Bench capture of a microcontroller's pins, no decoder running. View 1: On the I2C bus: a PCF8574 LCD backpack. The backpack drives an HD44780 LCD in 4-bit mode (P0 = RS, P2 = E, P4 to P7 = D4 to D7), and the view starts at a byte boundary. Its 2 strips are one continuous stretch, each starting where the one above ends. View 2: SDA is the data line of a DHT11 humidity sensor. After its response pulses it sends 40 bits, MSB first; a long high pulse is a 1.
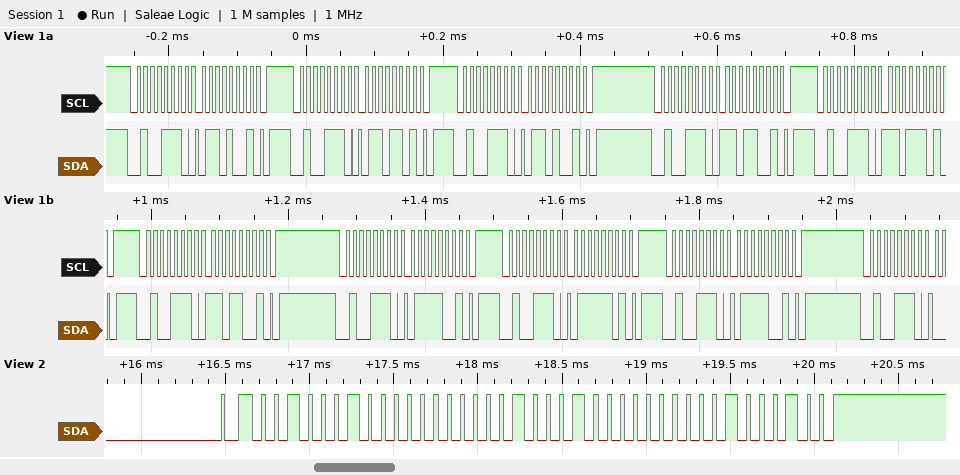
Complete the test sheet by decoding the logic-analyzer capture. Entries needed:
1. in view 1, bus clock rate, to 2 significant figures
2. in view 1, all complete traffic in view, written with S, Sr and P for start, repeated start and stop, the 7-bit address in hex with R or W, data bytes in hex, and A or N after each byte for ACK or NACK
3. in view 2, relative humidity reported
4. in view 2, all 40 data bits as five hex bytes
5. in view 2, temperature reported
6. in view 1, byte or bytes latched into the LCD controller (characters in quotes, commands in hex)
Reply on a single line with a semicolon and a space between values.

100 kHz; S 27W A 69 A P S 27W A 6D A P S 27W A 69 A P S 27W A D9 A P S 27W A DD A P S 27W A D9 A P S 27W A 79 A P S 27W A 7D A P S 27W A 79 A P S 27W A; 34 %; 22 00 22 00 44; 34.0 °C; 'm'
